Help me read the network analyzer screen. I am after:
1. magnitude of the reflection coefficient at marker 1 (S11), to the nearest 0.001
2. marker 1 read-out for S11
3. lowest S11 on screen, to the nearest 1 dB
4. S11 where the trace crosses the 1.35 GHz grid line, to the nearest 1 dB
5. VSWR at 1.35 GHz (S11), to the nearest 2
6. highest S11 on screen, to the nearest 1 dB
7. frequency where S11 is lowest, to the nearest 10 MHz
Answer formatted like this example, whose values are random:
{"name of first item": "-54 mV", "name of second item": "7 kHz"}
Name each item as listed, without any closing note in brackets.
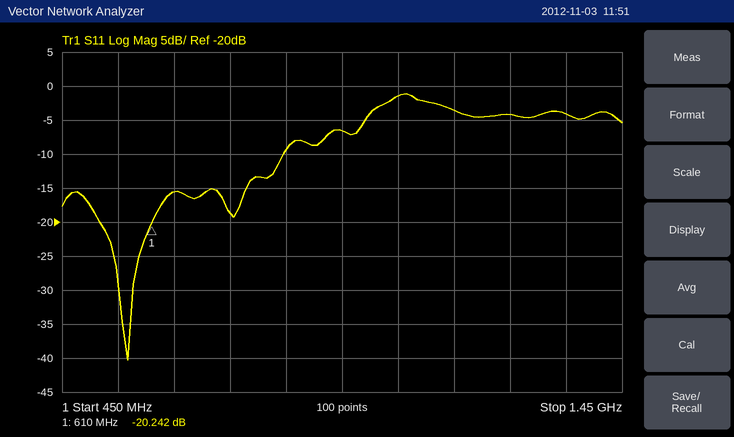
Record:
{"magnitude of the reflection coefficient at marker 1 (S11), to the nearest 0.001": "0.097", "marker 1 read-out for S11": "-20.242 dB", "lowest S11 on screen, to the nearest 1 dB": "-40 dB", "S11 where the trace crosses the 1.35 GHz grid line, to the nearest 1 dB": "-4 dB", "VSWR at 1.35 GHz (S11), to the nearest 2": "4", "highest S11 on screen, to the nearest 1 dB": "-1 dB", "frequency where S11 is lowest, to the nearest 10 MHz": "570 MHz"}
